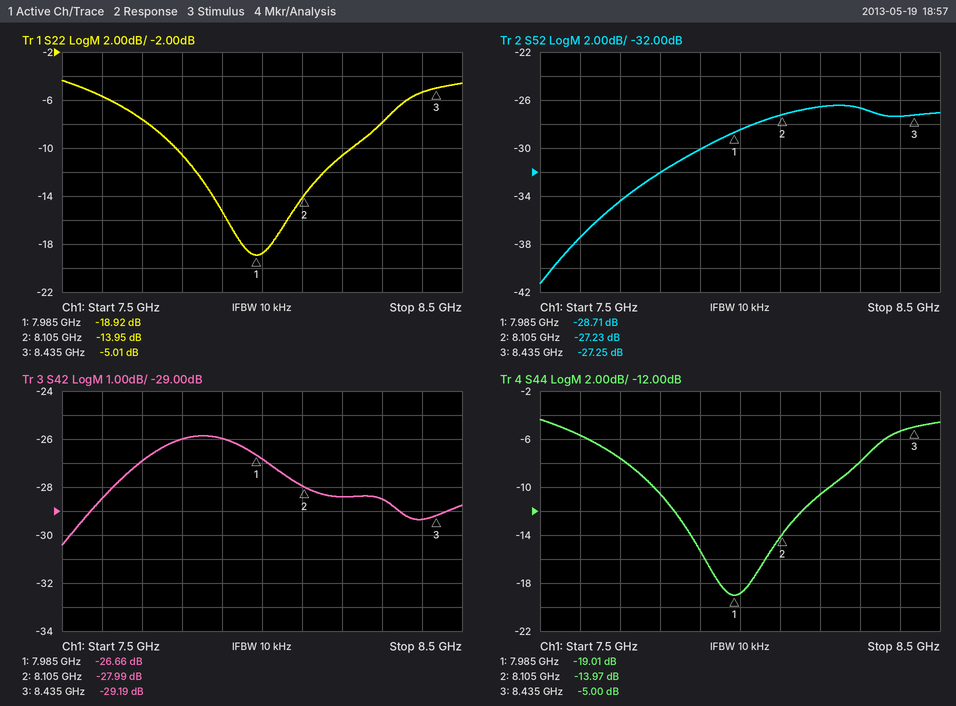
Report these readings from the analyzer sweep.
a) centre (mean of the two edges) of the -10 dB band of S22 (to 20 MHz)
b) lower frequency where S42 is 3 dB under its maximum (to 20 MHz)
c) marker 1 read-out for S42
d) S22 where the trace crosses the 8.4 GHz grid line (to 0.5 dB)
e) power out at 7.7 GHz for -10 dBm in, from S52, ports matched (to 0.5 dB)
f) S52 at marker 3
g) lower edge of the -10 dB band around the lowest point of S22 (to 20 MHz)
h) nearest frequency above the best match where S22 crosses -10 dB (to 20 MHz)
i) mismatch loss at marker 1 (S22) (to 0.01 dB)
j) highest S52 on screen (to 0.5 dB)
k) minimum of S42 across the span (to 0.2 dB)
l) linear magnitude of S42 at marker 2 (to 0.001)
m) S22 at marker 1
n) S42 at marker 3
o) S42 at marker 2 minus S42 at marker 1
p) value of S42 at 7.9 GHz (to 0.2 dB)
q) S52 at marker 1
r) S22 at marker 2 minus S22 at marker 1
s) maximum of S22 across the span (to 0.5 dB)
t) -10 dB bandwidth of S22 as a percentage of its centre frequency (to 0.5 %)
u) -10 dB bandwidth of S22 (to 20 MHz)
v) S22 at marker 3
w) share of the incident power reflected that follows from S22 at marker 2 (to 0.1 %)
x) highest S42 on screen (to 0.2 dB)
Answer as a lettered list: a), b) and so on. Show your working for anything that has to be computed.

a) 8.00 GHz
b) 7.58 GHz
c) -26.66 dB
d) -5.5 dB
e) -10 dBm + (-34.5 dB) = -44.5 dBm
f) -27.25 dB
g) 7.78 GHz
h) 8.22 GHz
i) −10 log10(1 − 10^(-18.92/10)) ≈ 0.06 dB
j) -26.5 dB
k) -30.4 dB
l) 10^(-27.99/20) ≈ 0.040
m) -18.92 dB
n) -29.19 dB
o) -27.99 − (-26.66) = -1.33 dB
p) -26.0 dB
q) -28.71 dB
r) -13.95 − (-18.92) = 4.97 dB
s) -4.5 dB
t) 440 MHz / 8 GHz ≈ 5.5 %
u) 8.22 GHz − 7.78 GHz = 440 MHz
v) -5.01 dB
w) 10^(-13.95/10) ≈ 4.0 %
x) -25.8 dB
